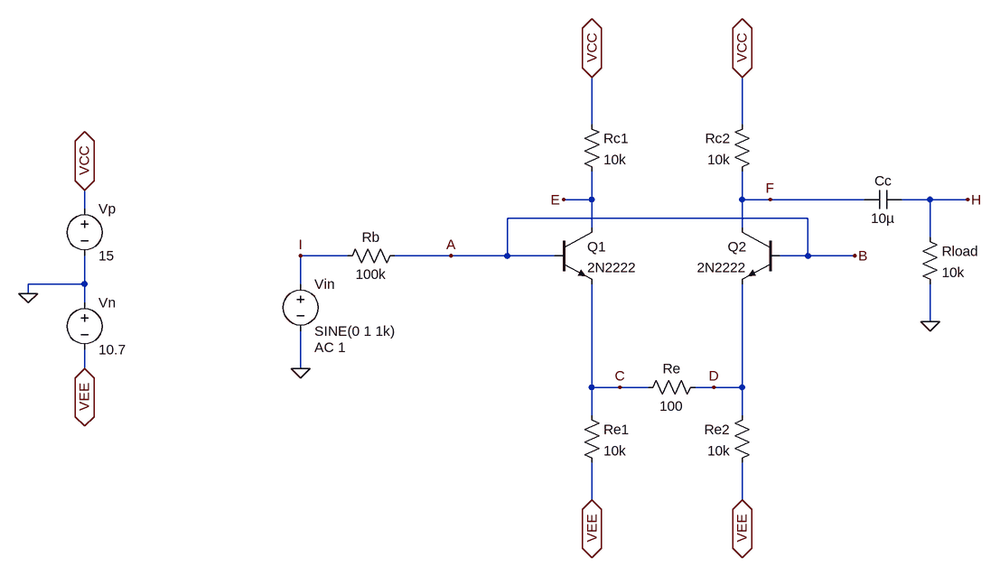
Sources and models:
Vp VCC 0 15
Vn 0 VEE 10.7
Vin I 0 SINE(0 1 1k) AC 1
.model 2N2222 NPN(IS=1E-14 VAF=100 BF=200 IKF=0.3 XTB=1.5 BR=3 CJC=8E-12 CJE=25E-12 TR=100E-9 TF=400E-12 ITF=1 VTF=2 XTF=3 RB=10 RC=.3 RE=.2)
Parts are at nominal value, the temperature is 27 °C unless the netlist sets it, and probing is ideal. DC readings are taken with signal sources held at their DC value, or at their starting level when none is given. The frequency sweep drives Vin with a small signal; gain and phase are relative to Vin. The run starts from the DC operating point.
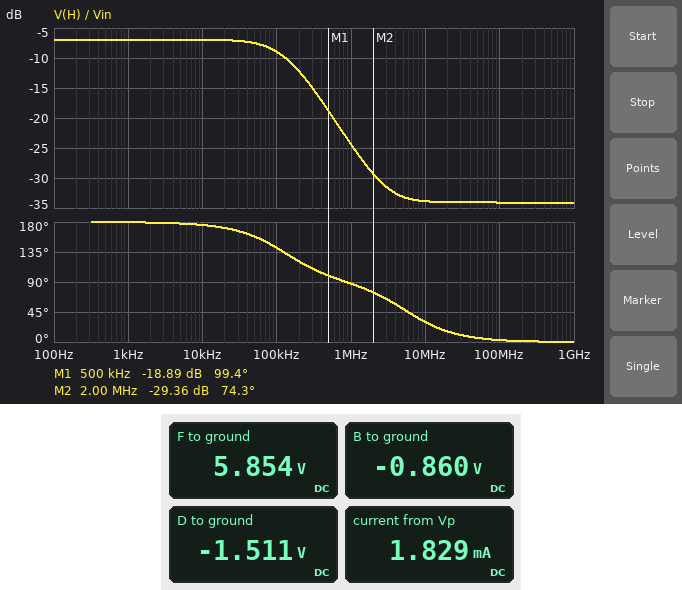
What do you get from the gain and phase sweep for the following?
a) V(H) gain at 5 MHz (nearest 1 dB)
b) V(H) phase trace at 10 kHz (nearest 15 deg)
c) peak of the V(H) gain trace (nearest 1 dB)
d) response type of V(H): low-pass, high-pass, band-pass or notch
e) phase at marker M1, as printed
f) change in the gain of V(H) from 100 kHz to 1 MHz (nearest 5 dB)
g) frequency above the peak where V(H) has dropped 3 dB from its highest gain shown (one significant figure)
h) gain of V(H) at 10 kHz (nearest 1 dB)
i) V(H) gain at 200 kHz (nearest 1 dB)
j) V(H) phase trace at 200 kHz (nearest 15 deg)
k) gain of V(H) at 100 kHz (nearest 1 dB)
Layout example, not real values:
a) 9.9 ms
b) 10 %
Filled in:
a) -33 dB
b) 180 deg
c) -7 dB
d) low-pass
e) 99.4 deg
f) -15 dB
g) 100 kHz
h) -7 dB
i) -12 dB
j) 120 deg
k) -9 dB
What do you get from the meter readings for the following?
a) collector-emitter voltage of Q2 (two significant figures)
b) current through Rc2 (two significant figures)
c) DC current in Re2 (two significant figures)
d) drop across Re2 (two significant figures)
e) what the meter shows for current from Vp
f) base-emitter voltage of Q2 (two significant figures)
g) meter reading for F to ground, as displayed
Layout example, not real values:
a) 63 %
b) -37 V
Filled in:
a) 7.4 V
b) 910 µA
c) 920 µA
d) 9.2 V
e) 1.829 mA
f) 650 mV
g) 5.854 V
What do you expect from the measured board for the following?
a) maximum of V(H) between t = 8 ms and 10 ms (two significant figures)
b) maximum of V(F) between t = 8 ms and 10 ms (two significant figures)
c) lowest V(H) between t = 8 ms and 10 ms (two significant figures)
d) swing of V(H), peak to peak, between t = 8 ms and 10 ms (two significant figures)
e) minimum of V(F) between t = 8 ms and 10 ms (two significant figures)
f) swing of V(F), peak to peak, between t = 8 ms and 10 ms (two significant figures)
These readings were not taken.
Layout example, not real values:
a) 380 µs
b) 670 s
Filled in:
a) 450 mV
b) 6.3 V
c) -450 mV
d) 900 mV
e) 5.4 V
f) 900 mV
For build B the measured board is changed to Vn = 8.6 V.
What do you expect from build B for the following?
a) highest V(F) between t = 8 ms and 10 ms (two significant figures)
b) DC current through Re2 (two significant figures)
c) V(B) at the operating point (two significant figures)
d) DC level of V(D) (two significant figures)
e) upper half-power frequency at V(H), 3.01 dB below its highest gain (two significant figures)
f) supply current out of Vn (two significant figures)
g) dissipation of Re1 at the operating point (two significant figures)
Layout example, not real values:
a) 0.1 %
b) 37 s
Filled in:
a) 8.2 V
b) 730 µA
c) -670 mV
d) -1.3 V
e) 140 kHz
f) 1.5 mA
g) 5.3 mW
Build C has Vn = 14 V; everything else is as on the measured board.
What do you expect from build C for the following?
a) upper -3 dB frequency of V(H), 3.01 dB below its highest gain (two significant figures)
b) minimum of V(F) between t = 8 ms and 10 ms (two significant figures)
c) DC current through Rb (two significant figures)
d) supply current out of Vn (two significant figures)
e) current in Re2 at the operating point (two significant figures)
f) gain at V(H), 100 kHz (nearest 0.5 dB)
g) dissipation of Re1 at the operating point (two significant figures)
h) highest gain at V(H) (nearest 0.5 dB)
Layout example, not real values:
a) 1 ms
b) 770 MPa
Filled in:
a) 110 kHz
b) 2.4 V
c) 12 µA
d) 2.4 mA
e) 1.2 mA
f) -9.5 dB
g) 15 mW
h) -7.0 dB
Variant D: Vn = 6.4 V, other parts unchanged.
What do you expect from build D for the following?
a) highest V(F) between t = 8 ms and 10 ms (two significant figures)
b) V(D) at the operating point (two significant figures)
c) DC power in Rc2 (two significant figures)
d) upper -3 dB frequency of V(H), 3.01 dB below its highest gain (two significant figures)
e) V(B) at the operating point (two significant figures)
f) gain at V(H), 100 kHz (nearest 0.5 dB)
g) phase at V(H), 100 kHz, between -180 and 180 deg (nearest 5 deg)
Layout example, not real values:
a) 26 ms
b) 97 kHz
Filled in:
a) 10 V
b) -1.1 V
c) 2.8 mW
d) 140 kHz
e) -480 mV
f) -8.5 dB
g) 145 deg
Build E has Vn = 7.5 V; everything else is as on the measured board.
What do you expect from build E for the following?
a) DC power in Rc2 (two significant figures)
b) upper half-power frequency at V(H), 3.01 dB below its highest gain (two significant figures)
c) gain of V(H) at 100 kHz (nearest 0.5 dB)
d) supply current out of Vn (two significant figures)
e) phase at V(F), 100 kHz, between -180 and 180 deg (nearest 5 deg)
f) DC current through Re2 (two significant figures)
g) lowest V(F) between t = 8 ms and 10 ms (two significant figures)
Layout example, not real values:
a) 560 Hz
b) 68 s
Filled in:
a) 3.9 mW
b) 140 kHz
c) -8.5 dB
d) 1.3 mA
e) 145 deg
f) 630 µA
g) 8.3 V
